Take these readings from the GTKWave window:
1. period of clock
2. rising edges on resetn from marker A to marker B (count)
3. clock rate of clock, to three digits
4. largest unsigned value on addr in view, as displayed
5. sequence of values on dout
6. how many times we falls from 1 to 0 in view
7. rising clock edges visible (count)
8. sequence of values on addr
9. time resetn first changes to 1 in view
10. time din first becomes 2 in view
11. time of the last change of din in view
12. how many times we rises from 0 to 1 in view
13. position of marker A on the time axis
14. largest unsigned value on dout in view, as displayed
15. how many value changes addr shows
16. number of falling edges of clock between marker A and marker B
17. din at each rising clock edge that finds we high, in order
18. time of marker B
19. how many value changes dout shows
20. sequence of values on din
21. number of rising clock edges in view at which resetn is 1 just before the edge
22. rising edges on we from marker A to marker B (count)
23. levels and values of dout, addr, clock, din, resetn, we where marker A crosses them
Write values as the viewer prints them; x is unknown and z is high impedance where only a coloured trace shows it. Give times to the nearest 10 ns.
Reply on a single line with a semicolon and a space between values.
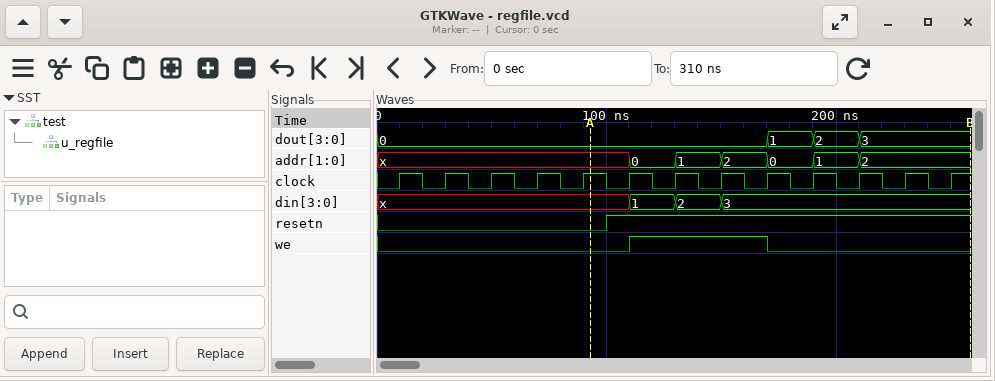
20 ns; 1; 50.0 MHz; 2; 0, 1, 2, 3; 1; 13; x, 0, 1, 2, 0, 1, 2; 100 ns; 130 ns; 150 ns; 1; 90 ns; 3; 6; 8; 1, 2, 3; 260 ns; 3; x, 1, 2, 3; 8; 1; dout=0, addr=x, clock=1, din=x, resetn=0, we=0
